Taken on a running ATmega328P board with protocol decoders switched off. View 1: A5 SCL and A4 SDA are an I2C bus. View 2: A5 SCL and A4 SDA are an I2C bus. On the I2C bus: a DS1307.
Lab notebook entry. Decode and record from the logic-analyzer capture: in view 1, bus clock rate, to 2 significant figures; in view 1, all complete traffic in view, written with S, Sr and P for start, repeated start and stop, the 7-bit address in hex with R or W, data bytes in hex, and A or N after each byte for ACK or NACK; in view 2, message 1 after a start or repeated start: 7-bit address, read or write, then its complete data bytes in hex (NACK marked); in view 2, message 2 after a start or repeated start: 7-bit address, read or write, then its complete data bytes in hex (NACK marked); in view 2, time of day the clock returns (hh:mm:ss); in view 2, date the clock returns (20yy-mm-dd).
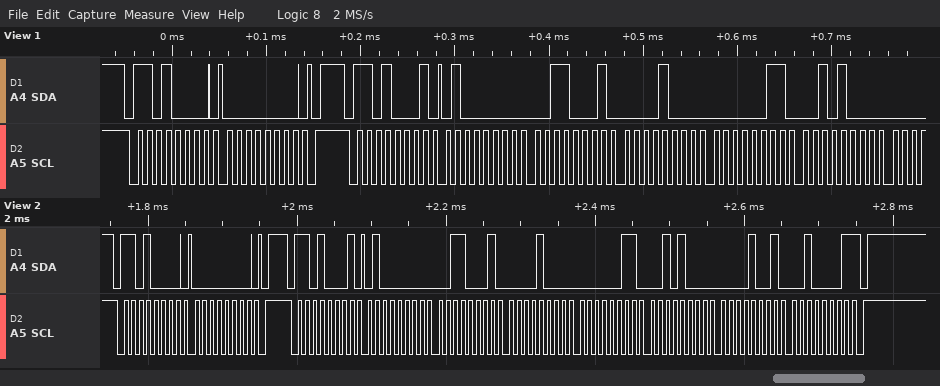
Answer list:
100 kHz
S 68W A 00 A P S 68R A 40 A 31 A 08 A 03 A 28 A
0x68 write: 00
0x68 read: 40 31 08 03 28 09 21 NACK
08:31:40
2021-09-28
